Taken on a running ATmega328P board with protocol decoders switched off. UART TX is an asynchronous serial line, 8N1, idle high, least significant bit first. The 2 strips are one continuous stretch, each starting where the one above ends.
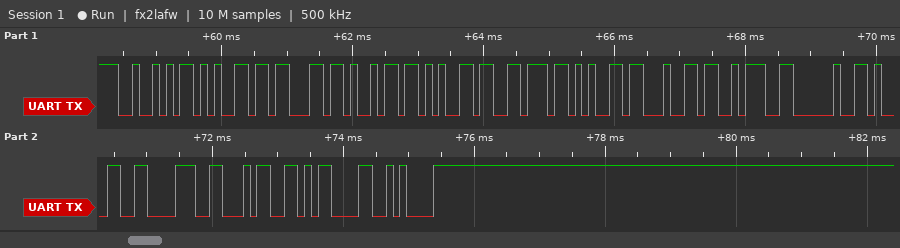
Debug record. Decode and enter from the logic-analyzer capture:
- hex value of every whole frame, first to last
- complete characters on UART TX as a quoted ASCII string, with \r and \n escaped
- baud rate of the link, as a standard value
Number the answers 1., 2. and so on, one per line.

1. 52 65 63 69 65 76 65 64 3A 20 31 38 34 0D 0A
2. "Recieved: 184\r\n"
3. 9600 baud
